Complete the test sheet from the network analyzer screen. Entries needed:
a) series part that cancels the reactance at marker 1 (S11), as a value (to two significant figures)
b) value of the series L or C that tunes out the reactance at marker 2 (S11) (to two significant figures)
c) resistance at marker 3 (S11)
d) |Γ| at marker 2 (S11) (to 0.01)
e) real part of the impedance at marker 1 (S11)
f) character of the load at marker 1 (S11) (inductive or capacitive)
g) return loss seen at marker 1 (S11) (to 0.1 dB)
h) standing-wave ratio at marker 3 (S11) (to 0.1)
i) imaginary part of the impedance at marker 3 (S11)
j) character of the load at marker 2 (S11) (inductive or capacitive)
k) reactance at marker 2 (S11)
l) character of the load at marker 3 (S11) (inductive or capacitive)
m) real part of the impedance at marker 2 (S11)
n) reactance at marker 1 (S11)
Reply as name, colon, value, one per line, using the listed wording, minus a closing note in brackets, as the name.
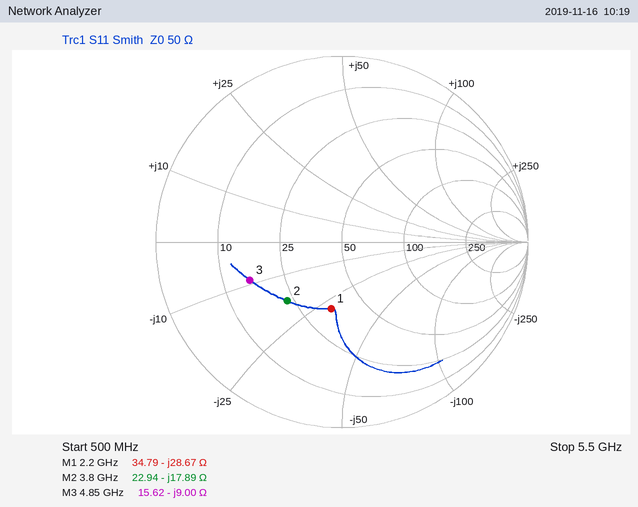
series part that cancels the reactance at marker 1 (S11), as a value: 2.1 nH
value of the series L or C that tunes out the reactance at marker 2 (S11): 750 pH
resistance at marker 3: 15.62 Ω
|Γ| at marker 2 (S11): 0.43
real part of the impedance at marker 1: 34.79 Ω
character of the load at marker 1 (S11): capacitive
return loss seen at marker 1 (S11): 8.8 dB
standing-wave ratio at marker 3 (S11): 3.3
imaginary part of the impedance at marker 3: -9.00 Ω
character of the load at marker 2 (S11): capacitive
reactance at marker 2: -17.89 Ω
character of the load at marker 3 (S11): capacitive
real part of the impedance at marker 2: 22.94 Ω
reactance at marker 1: -28.67 Ω
